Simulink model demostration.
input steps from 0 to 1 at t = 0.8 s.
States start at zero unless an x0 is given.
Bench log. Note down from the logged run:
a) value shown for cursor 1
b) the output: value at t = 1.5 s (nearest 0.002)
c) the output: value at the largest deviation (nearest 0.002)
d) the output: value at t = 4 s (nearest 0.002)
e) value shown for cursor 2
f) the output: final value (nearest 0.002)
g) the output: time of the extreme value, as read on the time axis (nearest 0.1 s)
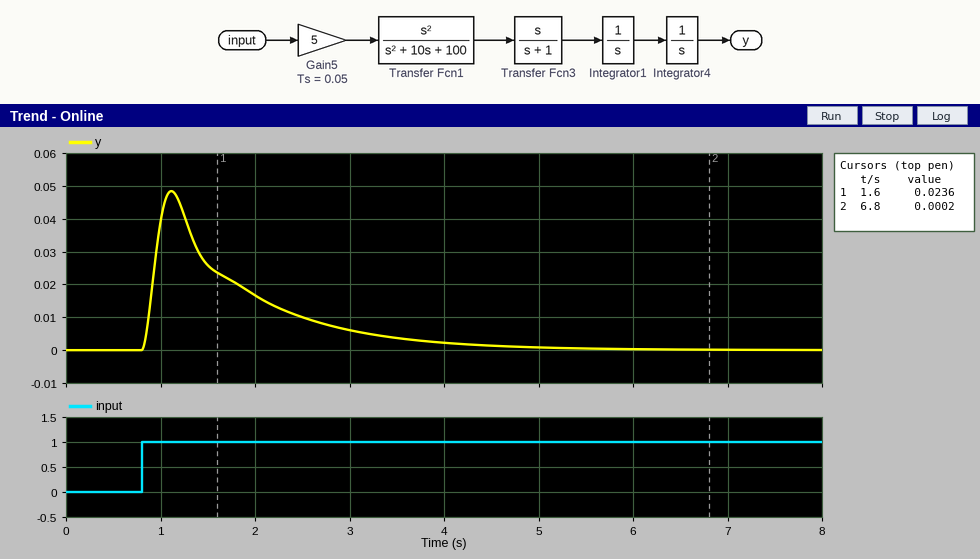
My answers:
0.0236
0.026
0.048
0.002
0.0002
0.000
1.1 s
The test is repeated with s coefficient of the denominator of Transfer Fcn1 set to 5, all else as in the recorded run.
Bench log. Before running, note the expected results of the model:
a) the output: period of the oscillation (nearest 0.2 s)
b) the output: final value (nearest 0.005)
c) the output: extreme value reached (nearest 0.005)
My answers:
0.6 s
0.000
0.060
